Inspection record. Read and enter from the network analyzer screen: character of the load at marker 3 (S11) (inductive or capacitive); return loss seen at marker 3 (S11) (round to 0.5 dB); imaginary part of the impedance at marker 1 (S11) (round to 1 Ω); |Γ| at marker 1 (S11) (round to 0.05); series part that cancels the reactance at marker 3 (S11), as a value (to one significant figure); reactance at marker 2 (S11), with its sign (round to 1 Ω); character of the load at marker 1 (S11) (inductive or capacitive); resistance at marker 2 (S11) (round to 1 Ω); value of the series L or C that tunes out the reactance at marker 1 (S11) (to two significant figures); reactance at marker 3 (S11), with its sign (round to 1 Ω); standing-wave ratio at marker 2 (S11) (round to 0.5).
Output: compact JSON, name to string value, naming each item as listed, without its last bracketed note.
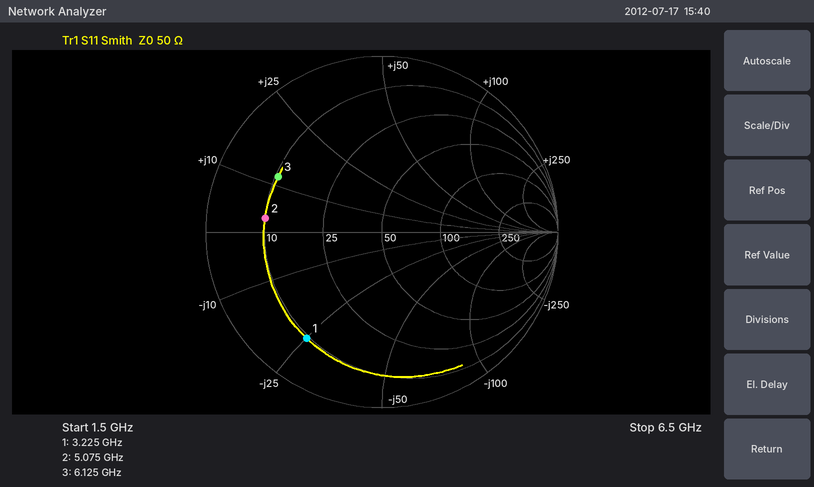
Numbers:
{"character of the load at marker 3 (S11)": "inductive", "return loss seen at marker 3 (S11)": "3.5 dB", "imaginary part of the impedance at marker 1 (S11)": "-25 Ω", "|Γ| at marker 1 (S11)": "0.75", "series part that cancels the reactance at marker 3 (S11), as a value": "2 pF", "reactance at marker 2 (S11), with its sign": "+3 Ω", "character of the load at marker 1 (S11)": "capacitive", "resistance at marker 2 (S11)": "10 Ω", "value of the series L or C that tunes out the reactance at marker 1 (S11)": "1.2 nH", "reactance at marker 3 (S11), with its sign": "+12 Ω", "standing-wave ratio at marker 2 (S11)": "5.0"}
